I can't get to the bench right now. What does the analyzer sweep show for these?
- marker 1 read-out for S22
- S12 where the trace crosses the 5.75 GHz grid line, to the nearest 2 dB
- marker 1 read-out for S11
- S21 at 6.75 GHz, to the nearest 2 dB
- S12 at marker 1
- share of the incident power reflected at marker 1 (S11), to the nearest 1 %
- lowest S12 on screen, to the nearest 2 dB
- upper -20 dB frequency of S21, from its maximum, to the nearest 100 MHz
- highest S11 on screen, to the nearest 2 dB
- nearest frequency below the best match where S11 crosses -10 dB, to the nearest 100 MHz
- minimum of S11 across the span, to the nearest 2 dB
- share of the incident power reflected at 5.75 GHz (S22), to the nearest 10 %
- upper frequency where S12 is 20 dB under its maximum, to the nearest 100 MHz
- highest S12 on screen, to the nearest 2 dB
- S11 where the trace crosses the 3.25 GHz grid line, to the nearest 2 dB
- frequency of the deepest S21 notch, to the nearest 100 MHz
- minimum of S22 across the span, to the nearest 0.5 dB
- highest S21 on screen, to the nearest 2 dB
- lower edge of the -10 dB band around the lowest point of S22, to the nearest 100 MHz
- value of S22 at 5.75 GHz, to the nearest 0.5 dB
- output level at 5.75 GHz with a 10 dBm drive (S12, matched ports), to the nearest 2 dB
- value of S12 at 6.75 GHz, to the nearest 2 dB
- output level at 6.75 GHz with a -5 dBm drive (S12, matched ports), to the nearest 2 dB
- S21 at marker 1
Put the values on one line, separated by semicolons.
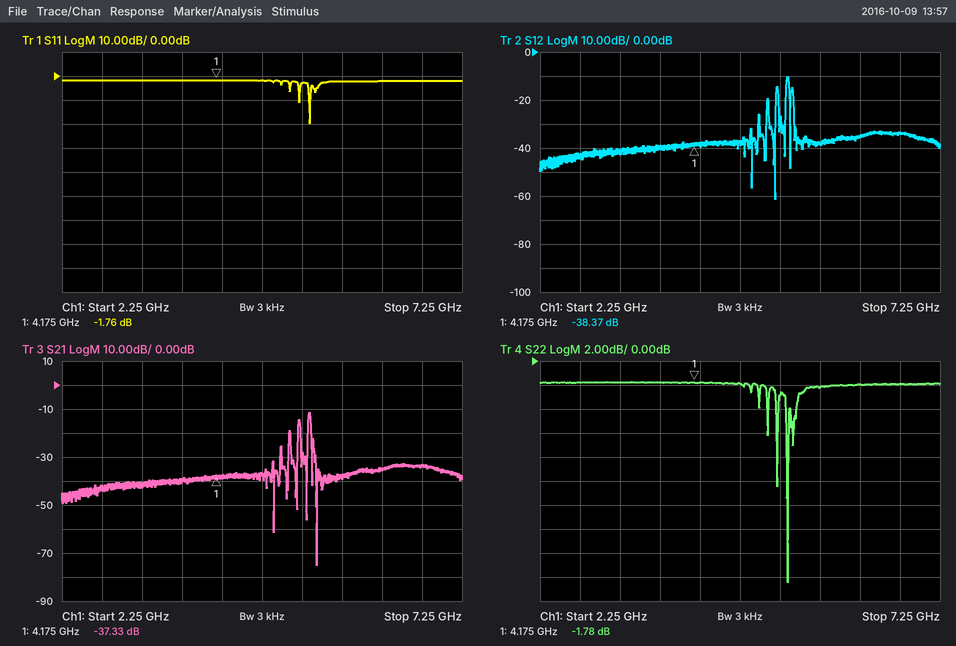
-1.78 dB; -38 dB; -1.76 dB; -34 dB; -38.37 dB; 67 %; -62 dB; 5.4 GHz; -2 dB; 5.3 GHz; -20 dB; 60 %; 5.4 GHz; -10 dB; -2 dB; 5.4 GHz; -18.5 dB; -12 dB; 5.3 GHz; -2.0 dB; -28 dBm; -34 dB; -38 dBm; -37.33 dB
